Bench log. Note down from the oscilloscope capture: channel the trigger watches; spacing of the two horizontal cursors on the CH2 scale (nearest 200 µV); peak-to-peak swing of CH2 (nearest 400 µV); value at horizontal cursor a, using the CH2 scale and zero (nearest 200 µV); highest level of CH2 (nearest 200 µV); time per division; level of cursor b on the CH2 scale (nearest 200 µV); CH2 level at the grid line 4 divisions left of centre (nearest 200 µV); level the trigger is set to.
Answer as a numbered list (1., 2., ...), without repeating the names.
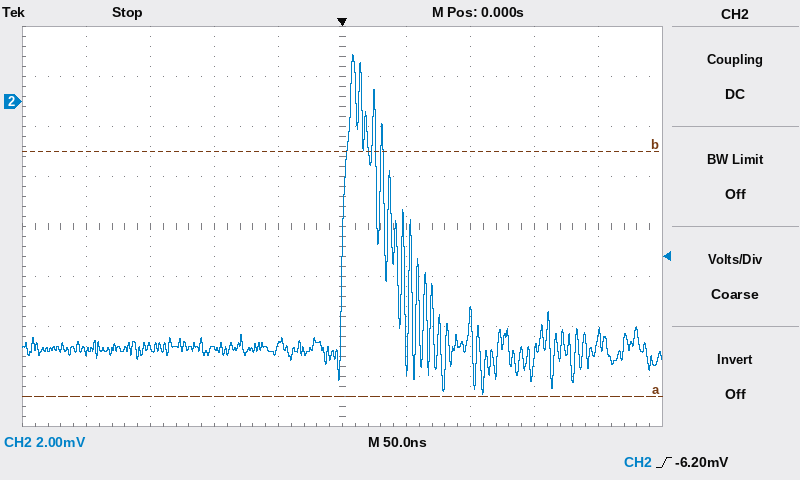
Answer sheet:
1. CH2
2. 9.8 mV
3. 13.6 mV
4. -11.8 mV
5. 1.8 mV
6. 50 ns
7. -2.0 mV
8. -10.0 mV
9. -6.20 mV
